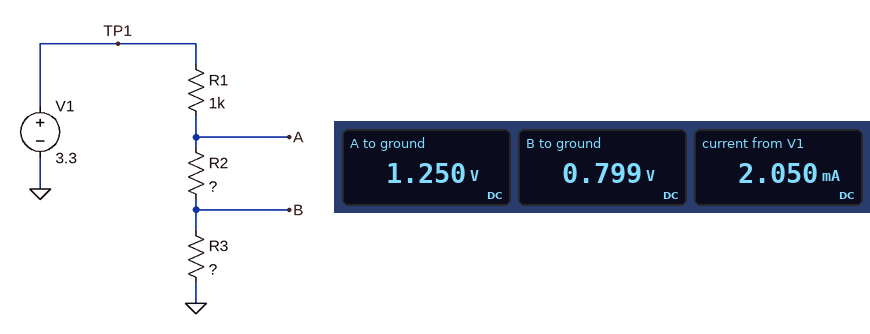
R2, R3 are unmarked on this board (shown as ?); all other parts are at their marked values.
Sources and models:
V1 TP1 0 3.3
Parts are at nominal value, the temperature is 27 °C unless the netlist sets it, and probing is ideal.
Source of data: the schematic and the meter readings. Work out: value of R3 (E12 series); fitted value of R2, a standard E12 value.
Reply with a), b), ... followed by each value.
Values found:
a) 390 Ω
b) 220 Ω
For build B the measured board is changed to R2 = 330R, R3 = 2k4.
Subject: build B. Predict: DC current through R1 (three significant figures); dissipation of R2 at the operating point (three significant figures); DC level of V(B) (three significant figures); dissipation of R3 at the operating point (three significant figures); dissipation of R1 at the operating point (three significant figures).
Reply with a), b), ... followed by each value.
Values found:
a) 885 µA
b) 258 µW
c) 2.12 V
d) 1.88 mW
e) 783 µW
